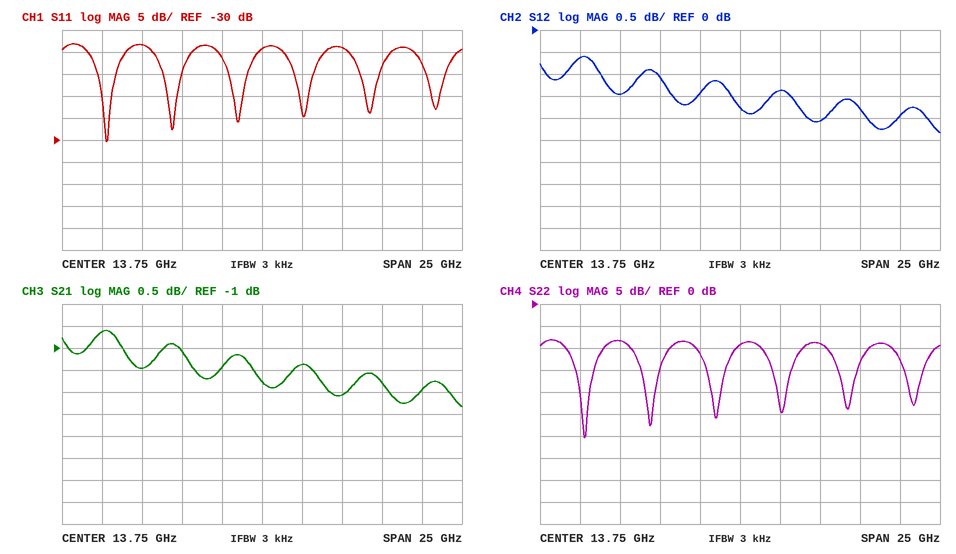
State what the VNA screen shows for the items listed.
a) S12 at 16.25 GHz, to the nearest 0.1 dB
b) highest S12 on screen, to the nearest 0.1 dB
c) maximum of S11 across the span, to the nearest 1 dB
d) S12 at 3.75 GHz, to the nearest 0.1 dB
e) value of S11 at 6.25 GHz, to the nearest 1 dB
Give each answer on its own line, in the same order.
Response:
-1.4 dB
-0.6 dB
-8 dB
-0.6 dB
-8 dB
